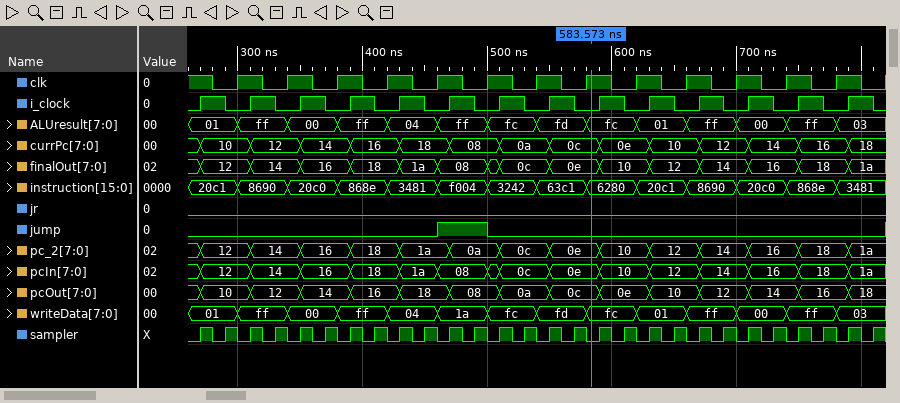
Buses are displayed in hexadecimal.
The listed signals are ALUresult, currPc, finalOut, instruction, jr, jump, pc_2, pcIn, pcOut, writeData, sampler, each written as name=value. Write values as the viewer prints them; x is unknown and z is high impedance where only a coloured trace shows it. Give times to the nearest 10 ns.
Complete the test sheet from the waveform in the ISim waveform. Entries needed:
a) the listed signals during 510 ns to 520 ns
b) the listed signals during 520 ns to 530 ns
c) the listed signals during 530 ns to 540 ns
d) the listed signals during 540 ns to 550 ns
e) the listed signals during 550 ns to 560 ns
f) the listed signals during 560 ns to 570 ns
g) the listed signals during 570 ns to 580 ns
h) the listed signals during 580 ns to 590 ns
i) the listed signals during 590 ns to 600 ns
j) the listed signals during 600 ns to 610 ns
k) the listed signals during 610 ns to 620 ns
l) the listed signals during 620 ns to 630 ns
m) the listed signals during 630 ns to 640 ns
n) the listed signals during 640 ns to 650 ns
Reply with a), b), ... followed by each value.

a) ALUresult=fc, currPc=0a, finalOut=0c, instruction=3242, jr=0, jump=0, pc_2=0c, pcIn=0c, pcOut=0a, writeData=fc, sampler=1
b) ALUresult=fc, currPc=0a, finalOut=0c, instruction=3242, jr=0, jump=0, pc_2=0c, pcIn=0c, pcOut=0a, writeData=fc, sampler=0
c) ALUresult=fc, currPc=0a, finalOut=0c, instruction=3242, jr=0, jump=0, pc_2=0c, pcIn=0c, pcOut=0a, writeData=fc, sampler=1
d) ALUresult=fd, currPc=0a, finalOut=0c, instruction=63c1, jr=0, jump=0, pc_2=0c, pcIn=0c, pcOut=0a, writeData=fd, sampler=0
e) ALUresult=fd, currPc=0c, finalOut=0e, instruction=63c1, jr=0, jump=0, pc_2=0e, pcIn=0e, pcOut=0c, writeData=fd, sampler=1
f) ALUresult=fd, currPc=0c, finalOut=0e, instruction=63c1, jr=0, jump=0, pc_2=0e, pcIn=0e, pcOut=0c, writeData=fd, sampler=0
g) ALUresult=fd, currPc=0c, finalOut=0e, instruction=63c1, jr=0, jump=0, pc_2=0e, pcIn=0e, pcOut=0c, writeData=fd, sampler=1
h) ALUresult=fc, currPc=0c, finalOut=0e, instruction=6280, jr=0, jump=0, pc_2=0e, pcIn=0e, pcOut=0c, writeData=fc, sampler=0
i) ALUresult=fc, currPc=0e, finalOut=10, instruction=6280, jr=0, jump=0, pc_2=10, pcIn=10, pcOut=0e, writeData=fc, sampler=1
j) ALUresult=fc, currPc=0e, finalOut=10, instruction=6280, jr=0, jump=0, pc_2=10, pcIn=10, pcOut=0e, writeData=fc, sampler=0
k) ALUresult=fc, currPc=0e, finalOut=10, instruction=6280, jr=0, jump=0, pc_2=10, pcIn=10, pcOut=0e, writeData=fc, sampler=1
l) ALUresult=01, currPc=0e, finalOut=10, instruction=20c1, jr=0, jump=0, pc_2=10, pcIn=10, pcOut=0e, writeData=01, sampler=0
m) ALUresult=01, currPc=10, finalOut=12, instruction=20c1, jr=0, jump=0, pc_2=12, pcIn=12, pcOut=10, writeData=01, sampler=1
n) ALUresult=01, currPc=10, finalOut=12, instruction=20c1, jr=0, jump=0, pc_2=12, pcIn=12, pcOut=10, writeData=01, sampler=0
